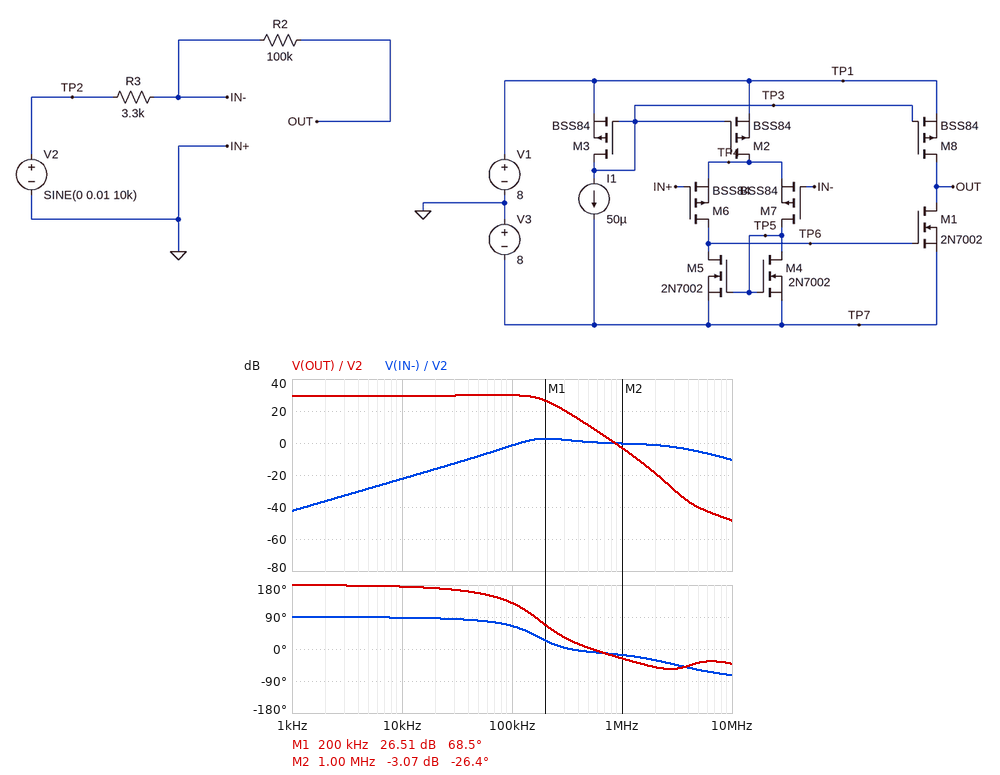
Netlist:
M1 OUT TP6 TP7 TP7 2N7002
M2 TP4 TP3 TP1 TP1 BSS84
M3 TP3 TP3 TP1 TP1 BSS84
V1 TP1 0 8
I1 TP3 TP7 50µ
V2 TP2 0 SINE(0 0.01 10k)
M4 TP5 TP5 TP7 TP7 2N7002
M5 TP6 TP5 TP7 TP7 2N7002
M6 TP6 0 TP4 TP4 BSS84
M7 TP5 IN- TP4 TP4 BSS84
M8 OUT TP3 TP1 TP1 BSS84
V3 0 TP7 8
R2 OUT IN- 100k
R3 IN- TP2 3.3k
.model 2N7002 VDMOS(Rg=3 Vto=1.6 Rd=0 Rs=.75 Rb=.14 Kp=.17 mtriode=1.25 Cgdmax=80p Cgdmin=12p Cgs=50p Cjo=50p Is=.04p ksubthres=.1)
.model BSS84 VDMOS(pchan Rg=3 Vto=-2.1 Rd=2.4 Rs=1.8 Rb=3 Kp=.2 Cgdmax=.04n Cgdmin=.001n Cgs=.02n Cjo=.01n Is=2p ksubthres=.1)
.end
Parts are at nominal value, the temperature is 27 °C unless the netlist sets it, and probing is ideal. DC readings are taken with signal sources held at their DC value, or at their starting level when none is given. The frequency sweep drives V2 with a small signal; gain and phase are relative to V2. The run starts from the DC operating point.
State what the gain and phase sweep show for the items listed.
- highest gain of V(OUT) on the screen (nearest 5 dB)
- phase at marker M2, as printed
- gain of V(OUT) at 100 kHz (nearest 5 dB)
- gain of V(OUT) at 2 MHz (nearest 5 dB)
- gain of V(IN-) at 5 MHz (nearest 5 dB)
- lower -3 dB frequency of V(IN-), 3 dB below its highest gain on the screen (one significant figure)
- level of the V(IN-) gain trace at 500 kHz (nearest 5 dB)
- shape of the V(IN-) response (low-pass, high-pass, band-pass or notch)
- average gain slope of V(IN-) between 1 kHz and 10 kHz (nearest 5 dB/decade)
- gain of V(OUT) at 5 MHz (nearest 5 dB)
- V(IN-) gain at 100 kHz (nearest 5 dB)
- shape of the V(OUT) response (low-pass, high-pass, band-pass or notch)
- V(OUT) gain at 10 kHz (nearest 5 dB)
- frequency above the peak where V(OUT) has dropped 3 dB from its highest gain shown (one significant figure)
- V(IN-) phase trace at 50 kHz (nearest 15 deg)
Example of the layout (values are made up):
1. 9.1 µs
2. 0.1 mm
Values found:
1. 30 dB
2. -26.4 deg
3. 30 dB
4. -20 dB
5. -5 dB
6. 100 kHz
7. 0 dB
8. band-pass
9. 20 dB/decade
10. -40 dB
11. 0 dB
12. low-pass
13. 30 dB
14. 200 kHz
15. 75 deg
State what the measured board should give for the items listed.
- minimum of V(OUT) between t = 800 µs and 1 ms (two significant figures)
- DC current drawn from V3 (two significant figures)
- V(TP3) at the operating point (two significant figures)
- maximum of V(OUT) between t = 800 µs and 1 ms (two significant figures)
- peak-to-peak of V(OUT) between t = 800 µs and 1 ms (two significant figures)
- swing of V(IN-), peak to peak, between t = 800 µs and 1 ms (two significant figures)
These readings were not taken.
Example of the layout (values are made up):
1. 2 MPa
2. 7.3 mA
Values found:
1. -300 mV
2. 150 µA
3. 6.0 V
4. 300 mV
5. 610 mV
6. 1.5 mV
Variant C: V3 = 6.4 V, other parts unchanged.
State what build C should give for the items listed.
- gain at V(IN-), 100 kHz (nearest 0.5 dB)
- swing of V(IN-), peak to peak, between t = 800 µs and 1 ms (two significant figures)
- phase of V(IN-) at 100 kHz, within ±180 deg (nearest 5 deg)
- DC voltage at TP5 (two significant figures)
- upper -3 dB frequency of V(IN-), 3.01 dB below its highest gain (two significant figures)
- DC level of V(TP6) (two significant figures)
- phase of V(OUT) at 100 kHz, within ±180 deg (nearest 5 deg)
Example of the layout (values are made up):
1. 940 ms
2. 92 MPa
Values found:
1. -1.0 dB
2. 1.6 mV
3. 60 deg
4. -5.0 V
5. 980 kHz
6. -4.9 V
7. 125 deg
